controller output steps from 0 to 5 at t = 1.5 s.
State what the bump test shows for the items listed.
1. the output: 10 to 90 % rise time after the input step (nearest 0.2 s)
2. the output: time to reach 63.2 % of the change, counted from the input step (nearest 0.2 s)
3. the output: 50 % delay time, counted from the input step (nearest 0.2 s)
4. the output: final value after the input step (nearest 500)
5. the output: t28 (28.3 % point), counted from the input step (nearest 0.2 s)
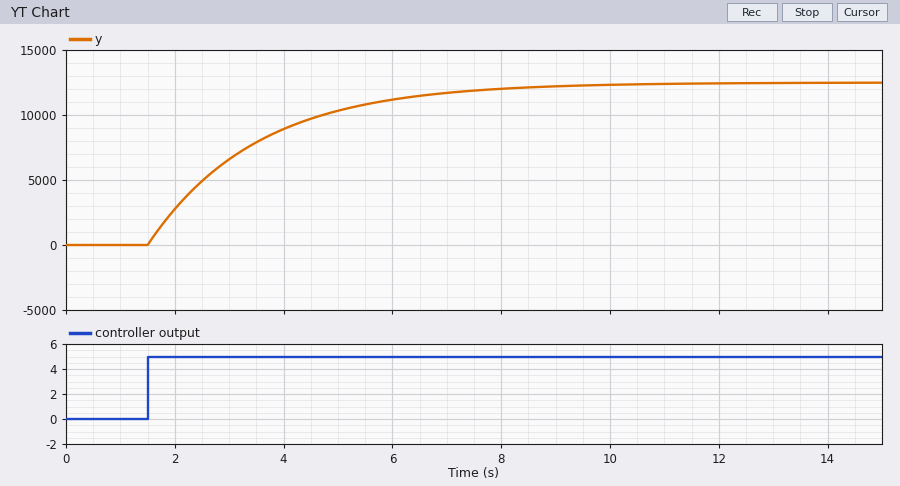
4.4 s
2.0 s
1.4 s
12500
0.6 s
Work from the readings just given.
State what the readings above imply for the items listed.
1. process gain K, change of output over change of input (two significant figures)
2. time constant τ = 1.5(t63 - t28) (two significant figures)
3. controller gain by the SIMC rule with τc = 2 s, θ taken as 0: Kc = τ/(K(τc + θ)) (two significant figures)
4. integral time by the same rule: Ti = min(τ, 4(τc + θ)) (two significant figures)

2500
2.1 s
0.00042
2.1 s
